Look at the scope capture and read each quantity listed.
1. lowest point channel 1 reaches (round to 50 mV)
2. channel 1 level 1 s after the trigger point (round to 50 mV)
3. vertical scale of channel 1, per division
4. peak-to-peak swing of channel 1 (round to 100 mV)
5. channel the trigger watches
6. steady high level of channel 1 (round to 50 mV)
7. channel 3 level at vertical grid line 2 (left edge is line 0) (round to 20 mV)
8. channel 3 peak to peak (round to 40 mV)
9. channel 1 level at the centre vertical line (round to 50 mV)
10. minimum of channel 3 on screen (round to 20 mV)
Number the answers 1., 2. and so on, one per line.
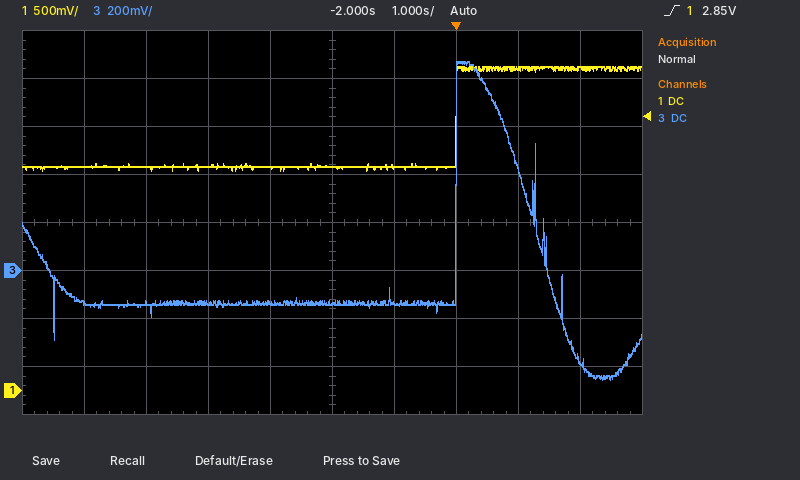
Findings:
1. 2.30 V
2. 3.35 V
3. 500 mV
4. 1.10 V
5. channel 1
6. 3.35 V
7. -140 mV
8. 1.32 V
9. 2.35 V
10. -460 mV
